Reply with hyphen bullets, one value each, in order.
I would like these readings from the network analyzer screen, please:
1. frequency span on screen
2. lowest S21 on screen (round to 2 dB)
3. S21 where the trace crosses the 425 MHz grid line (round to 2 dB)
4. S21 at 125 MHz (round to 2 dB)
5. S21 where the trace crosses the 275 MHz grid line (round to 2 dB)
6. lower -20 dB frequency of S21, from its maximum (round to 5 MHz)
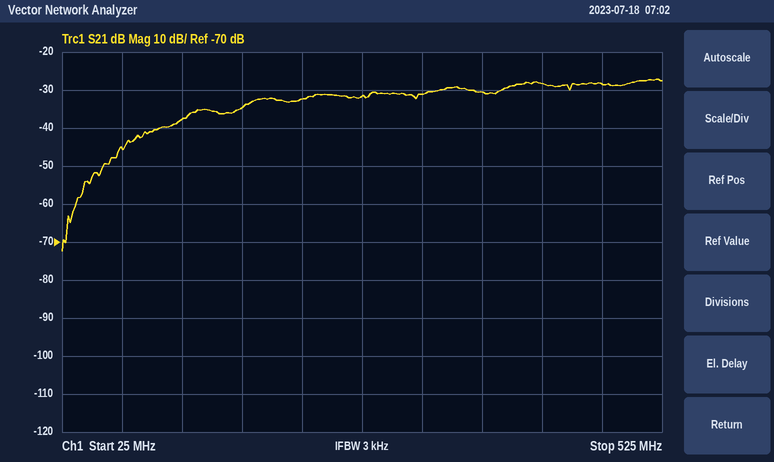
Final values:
- 500 MHz
- -72 dB
- -28 dB
- -38 dB
- -32 dB
- 70 MHz
